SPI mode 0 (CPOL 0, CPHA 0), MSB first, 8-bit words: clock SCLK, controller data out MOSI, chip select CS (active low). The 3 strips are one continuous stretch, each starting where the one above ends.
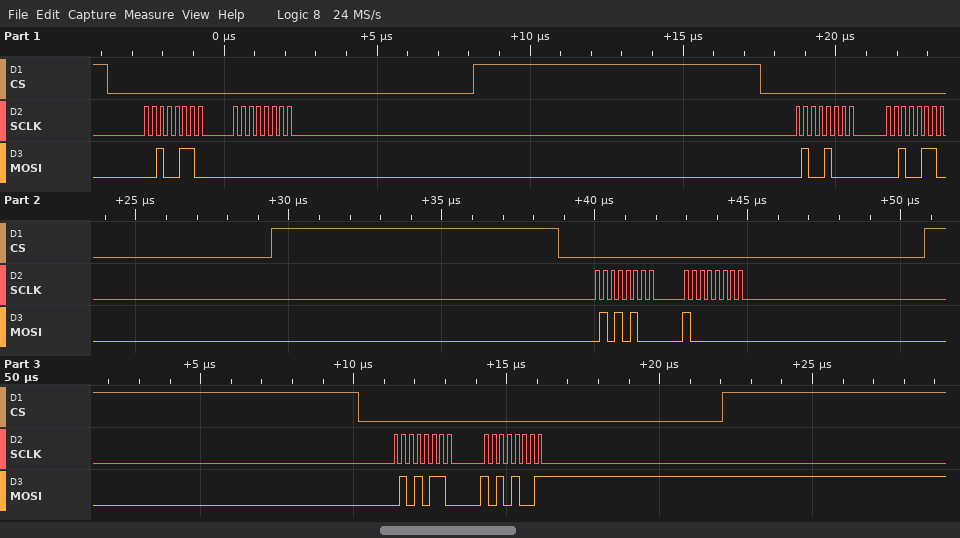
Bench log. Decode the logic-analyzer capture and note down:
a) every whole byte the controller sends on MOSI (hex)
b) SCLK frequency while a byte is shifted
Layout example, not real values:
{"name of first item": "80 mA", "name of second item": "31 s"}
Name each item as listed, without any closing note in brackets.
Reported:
{"every whole byte the controller sends on MOSI": "26 00 48 26 54 80 56 A9", "SCLK frequency while a byte is shifted": "4 MHz"}
